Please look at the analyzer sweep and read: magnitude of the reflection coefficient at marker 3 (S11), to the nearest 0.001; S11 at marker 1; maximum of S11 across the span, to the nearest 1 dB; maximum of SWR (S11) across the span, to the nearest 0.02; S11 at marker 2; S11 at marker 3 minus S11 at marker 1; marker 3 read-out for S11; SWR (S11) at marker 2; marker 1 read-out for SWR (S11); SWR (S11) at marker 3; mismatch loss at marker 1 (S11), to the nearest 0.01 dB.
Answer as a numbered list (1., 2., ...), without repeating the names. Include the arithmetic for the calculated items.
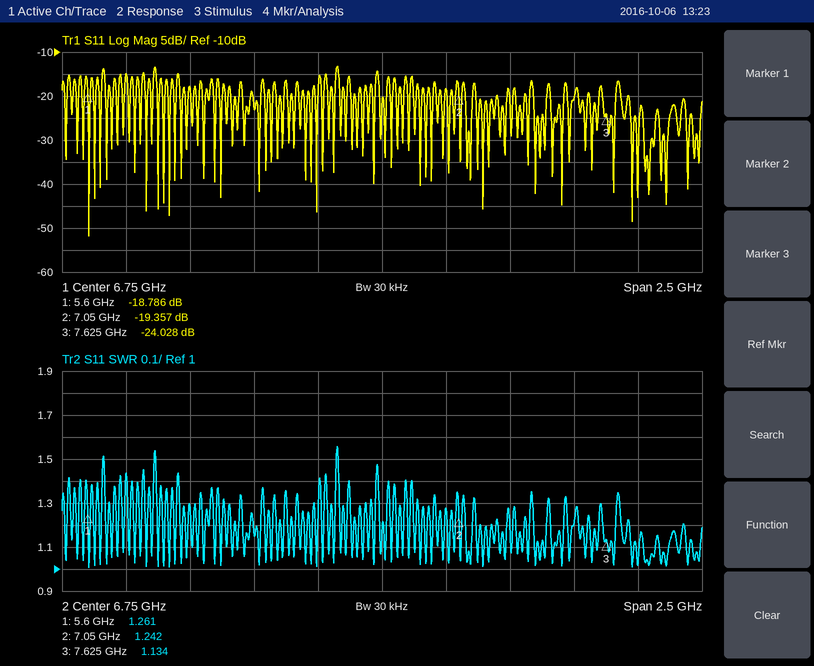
1. 10^(-24.028/20) ≈ 0.063
2. -18.786 dB
3. -13 dB
4. 1.56
5. -19.357 dB
6. -24.028 − (-18.786) = -5.242 dB
7. -24.028 dB
8. 1.242
9. 1.261
10. 1.134
11. −10 log10(1 − 10^(-18.786/10)) ≈ 0.06 dB
